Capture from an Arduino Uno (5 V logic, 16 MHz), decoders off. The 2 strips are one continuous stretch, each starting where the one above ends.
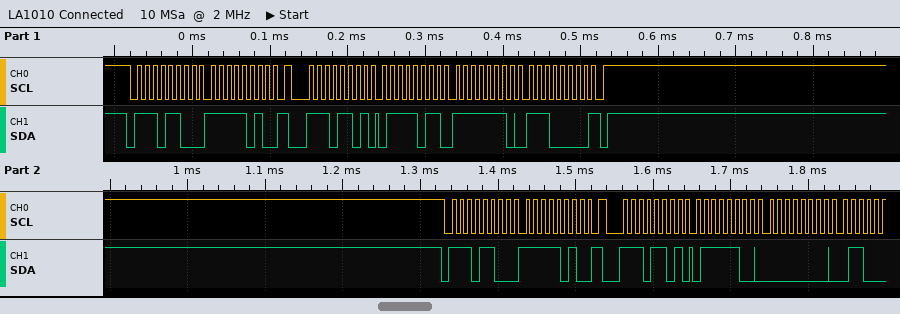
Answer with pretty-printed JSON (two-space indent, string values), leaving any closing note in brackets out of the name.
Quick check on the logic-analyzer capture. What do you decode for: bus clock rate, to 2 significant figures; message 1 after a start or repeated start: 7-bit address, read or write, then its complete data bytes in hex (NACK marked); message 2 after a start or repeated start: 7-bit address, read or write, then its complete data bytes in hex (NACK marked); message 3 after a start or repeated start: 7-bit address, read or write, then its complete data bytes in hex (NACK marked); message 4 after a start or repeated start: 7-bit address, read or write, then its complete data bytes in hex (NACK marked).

{
  "bus clock rate, to 2 significant figures": "100 kHz",
  "message 1 after a start or repeated start: 7-bit address, read or write, then its complete data bytes in hex": "0x76 write: FA",
  "message 2 after a start or repeated start: 7-bit address, read or write, then its complete data bytes in hex": "0x76 read: 7B FE E0 NACK",
  "message 3 after a start or repeated start: 7-bit address, read or write, then its complete data bytes in hex": "0x76 write: FA",
  "message 4 after a start or repeated start: 7-bit address, read or write, then its complete data bytes in hex": "0x76 read: 7C 00"
}
